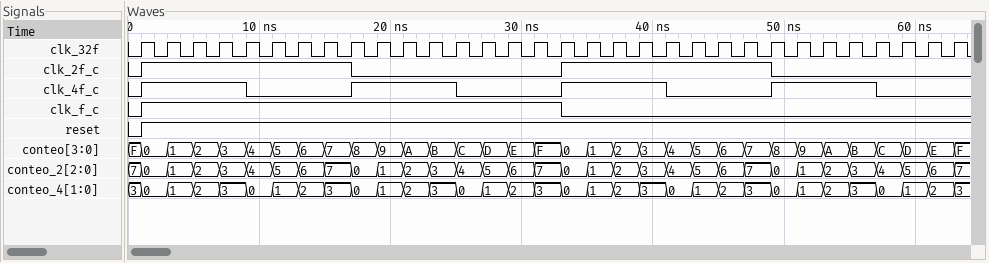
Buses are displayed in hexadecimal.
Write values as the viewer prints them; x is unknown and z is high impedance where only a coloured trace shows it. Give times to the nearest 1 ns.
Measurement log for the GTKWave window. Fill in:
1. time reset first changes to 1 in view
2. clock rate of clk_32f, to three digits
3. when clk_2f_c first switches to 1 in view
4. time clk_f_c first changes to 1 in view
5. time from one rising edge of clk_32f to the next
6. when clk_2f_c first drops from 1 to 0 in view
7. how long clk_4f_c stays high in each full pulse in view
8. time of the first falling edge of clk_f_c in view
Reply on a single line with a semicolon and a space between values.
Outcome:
1 ns; 500 MHz; 1 ns; 1 ns; 2 ns; 17 ns; 8 ns, 8 ns, 8 ns, 8 ns; 33 ns
